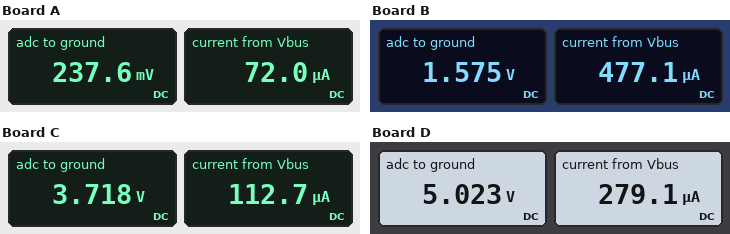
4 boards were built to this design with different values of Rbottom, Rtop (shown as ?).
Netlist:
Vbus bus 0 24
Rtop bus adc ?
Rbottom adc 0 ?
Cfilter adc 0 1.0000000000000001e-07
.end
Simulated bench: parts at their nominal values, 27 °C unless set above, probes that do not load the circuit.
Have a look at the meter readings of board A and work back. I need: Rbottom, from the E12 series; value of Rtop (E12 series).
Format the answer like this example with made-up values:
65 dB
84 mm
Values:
3.3 kΩ
330 kΩ
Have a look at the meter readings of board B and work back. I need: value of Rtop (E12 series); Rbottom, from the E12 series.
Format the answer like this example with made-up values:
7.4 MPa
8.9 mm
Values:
47 kΩ
3.3 kΩ
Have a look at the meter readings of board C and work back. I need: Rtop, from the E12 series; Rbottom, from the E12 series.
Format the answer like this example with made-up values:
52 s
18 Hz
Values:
180 kΩ
33 kΩ
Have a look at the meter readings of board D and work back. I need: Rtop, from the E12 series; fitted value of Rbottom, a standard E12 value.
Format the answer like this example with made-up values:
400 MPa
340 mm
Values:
68 kΩ
18 kΩ
